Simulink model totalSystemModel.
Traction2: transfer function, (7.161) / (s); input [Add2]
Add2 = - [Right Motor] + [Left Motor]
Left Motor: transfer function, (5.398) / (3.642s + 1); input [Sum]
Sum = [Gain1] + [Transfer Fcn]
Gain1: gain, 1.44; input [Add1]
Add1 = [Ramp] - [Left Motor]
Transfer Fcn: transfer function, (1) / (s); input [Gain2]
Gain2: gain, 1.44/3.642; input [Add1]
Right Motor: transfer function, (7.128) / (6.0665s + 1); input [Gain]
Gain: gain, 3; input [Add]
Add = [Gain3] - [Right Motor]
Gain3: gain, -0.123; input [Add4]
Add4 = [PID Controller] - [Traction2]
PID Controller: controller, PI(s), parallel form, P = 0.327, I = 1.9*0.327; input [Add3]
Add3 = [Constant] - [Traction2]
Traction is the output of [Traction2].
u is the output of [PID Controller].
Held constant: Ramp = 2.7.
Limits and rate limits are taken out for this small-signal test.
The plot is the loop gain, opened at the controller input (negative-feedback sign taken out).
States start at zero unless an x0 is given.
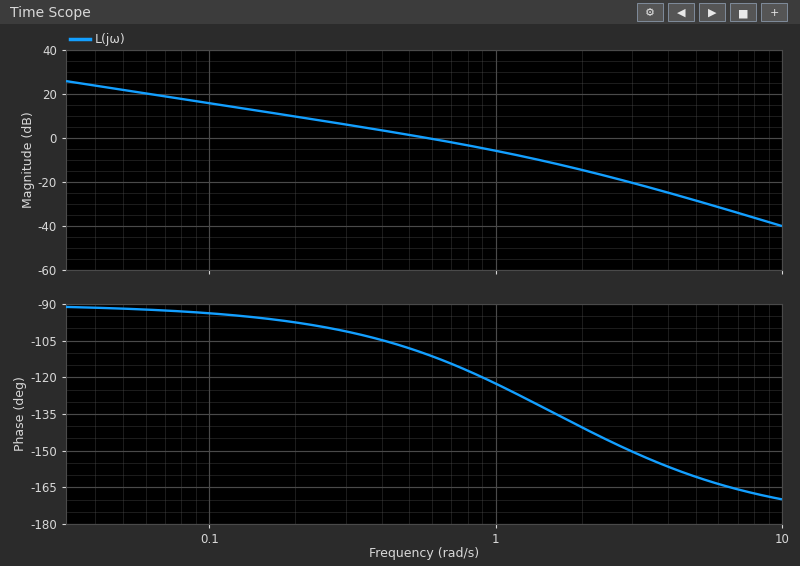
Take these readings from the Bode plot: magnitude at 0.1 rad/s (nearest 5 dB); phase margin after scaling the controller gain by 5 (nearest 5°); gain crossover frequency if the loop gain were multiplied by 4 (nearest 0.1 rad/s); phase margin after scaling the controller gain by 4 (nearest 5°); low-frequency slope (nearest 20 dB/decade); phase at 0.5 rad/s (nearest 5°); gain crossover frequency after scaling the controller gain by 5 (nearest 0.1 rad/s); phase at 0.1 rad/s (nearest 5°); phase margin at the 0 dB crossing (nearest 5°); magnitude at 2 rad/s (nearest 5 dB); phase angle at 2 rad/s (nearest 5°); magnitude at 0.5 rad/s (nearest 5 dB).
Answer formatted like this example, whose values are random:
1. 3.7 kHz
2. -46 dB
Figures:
1. 15 dB
2. 40°
3. 1.7 rad/s
4. 45°
5. -20 dB/decade
6. -110°
7. 1.9 rad/s
8. -95°
9. 70°
10. -15 dB
11. -140°
12. 0 dB
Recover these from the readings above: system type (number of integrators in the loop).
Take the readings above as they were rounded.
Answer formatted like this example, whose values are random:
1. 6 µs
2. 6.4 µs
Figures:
1. 1
